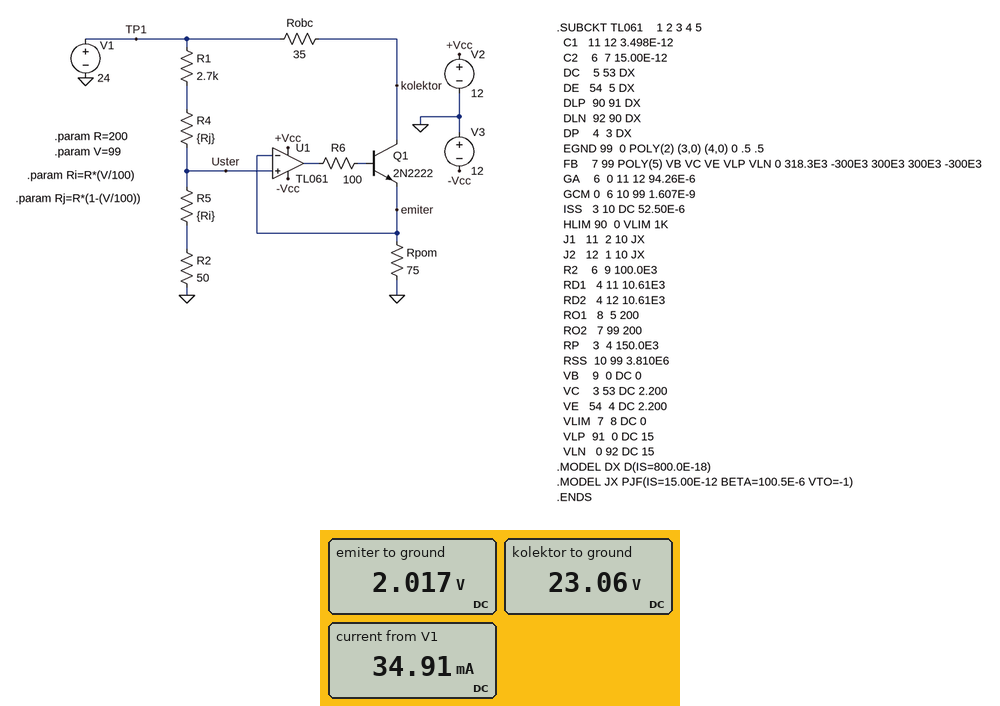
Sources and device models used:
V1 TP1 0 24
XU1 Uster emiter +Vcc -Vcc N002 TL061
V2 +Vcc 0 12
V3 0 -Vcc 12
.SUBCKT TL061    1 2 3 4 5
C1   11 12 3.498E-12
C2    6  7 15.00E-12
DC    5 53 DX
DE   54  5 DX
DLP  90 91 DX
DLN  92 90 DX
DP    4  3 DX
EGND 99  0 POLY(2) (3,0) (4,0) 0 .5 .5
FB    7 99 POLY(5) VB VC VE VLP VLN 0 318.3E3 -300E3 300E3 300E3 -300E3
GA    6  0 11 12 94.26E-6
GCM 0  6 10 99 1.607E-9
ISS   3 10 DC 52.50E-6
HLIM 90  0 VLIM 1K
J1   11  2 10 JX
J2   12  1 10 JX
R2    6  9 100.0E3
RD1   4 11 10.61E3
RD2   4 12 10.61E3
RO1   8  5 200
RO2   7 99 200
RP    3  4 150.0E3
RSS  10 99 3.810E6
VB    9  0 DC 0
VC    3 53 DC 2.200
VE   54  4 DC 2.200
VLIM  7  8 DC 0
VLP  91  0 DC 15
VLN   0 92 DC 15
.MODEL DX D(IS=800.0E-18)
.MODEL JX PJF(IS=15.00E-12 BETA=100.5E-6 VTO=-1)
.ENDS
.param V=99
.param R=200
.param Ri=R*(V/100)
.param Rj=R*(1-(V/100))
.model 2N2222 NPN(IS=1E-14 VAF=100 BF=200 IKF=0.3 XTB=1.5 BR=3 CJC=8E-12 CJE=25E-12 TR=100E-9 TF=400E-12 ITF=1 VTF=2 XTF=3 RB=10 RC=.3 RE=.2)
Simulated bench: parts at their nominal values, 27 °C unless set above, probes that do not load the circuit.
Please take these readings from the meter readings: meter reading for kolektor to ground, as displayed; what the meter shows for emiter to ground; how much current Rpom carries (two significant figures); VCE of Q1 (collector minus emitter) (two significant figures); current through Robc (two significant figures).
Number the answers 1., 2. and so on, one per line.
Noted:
1. 23.06 V
2. 2.017 V
3. 27 mA
4. 21 V
5. 27 mA
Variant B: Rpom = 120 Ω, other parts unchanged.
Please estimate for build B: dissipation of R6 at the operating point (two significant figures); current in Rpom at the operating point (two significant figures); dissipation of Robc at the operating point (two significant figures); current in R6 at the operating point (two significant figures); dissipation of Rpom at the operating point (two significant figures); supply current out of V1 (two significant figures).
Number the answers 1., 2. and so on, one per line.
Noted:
1. 530 nW
2. 17 mA
3. 9.8 mW
4. 73 µA
5. 34 mW
6. 25 mA
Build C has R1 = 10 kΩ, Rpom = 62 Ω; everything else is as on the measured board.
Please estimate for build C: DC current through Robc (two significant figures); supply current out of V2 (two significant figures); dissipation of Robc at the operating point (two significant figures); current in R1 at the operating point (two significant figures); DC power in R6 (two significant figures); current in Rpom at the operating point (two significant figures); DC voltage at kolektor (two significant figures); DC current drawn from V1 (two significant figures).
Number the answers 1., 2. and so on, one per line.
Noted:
1. 9.3 mA
2. 210 µA
3. 3.0 mW
4. 2.3 mA
5. 150 nW
6. 9.4 mA
7. 24 V
8. 12 mA
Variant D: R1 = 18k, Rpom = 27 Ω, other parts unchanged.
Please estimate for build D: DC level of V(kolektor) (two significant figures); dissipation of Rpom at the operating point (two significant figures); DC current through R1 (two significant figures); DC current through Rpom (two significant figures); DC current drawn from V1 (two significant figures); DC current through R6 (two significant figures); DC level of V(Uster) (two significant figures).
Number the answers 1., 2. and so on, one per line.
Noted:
1. 24 V
2. 3.9 mW
3. 1.3 mA
4. 12 mA
5. 13 mA
6. 51 µA
7. 330 mV
